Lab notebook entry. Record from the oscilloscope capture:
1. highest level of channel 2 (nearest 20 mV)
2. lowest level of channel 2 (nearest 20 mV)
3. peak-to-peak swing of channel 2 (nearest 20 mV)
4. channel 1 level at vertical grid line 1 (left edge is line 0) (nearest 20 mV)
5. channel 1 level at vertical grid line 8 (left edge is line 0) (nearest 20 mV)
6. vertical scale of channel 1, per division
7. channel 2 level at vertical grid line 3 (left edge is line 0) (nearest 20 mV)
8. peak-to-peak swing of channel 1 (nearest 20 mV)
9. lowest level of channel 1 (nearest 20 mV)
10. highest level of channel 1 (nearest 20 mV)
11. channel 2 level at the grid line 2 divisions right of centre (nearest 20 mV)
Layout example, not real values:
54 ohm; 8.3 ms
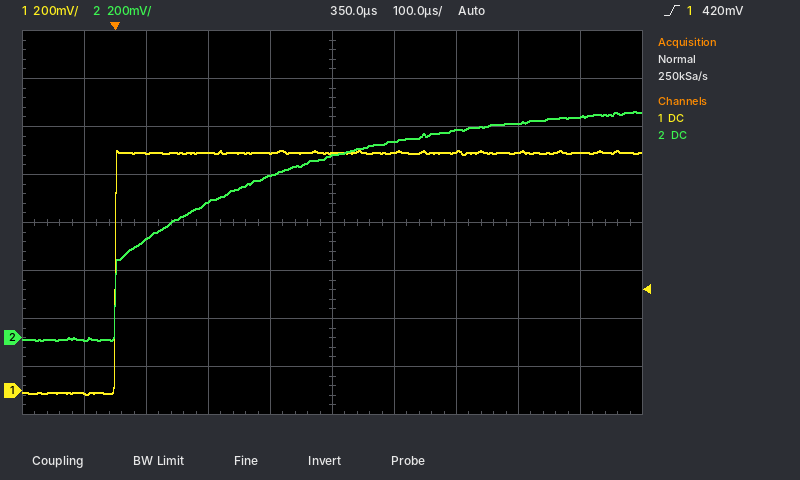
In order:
940 mV; -20 mV; 960 mV; -20 mV; 1.00 V; 200 mV; 560 mV; 1.02 V; -20 mV; 1.00 V; 860 mV
